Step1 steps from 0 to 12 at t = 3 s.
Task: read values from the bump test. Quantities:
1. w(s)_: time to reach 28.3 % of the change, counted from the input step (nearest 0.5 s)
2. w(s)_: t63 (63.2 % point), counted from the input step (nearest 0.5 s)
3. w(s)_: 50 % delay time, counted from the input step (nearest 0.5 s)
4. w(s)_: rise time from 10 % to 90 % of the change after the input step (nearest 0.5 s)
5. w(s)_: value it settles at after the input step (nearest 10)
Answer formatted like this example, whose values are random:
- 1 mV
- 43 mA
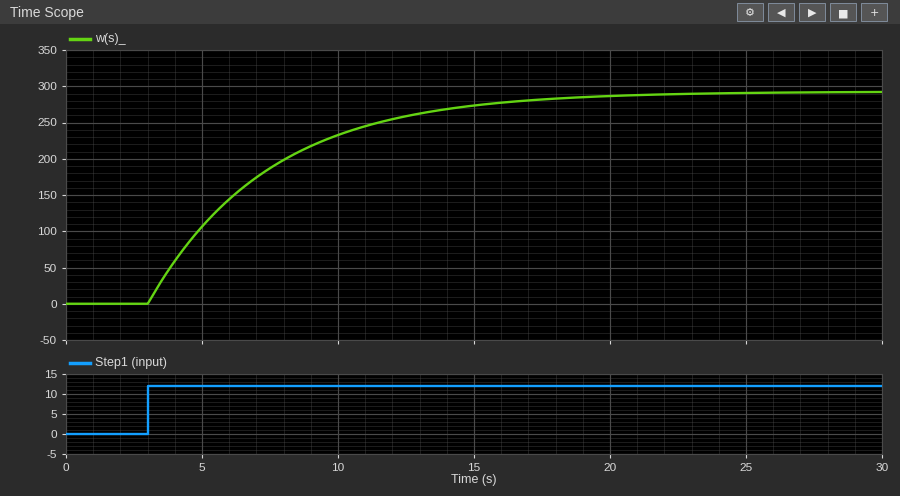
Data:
- 1.5 s
- 4.5 s
- 3.0 s
- 9.5 s
- 290
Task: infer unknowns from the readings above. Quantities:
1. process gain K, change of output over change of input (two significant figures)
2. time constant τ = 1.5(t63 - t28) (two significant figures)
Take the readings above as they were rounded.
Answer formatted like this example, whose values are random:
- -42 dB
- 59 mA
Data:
- 24
- 4.5 s
